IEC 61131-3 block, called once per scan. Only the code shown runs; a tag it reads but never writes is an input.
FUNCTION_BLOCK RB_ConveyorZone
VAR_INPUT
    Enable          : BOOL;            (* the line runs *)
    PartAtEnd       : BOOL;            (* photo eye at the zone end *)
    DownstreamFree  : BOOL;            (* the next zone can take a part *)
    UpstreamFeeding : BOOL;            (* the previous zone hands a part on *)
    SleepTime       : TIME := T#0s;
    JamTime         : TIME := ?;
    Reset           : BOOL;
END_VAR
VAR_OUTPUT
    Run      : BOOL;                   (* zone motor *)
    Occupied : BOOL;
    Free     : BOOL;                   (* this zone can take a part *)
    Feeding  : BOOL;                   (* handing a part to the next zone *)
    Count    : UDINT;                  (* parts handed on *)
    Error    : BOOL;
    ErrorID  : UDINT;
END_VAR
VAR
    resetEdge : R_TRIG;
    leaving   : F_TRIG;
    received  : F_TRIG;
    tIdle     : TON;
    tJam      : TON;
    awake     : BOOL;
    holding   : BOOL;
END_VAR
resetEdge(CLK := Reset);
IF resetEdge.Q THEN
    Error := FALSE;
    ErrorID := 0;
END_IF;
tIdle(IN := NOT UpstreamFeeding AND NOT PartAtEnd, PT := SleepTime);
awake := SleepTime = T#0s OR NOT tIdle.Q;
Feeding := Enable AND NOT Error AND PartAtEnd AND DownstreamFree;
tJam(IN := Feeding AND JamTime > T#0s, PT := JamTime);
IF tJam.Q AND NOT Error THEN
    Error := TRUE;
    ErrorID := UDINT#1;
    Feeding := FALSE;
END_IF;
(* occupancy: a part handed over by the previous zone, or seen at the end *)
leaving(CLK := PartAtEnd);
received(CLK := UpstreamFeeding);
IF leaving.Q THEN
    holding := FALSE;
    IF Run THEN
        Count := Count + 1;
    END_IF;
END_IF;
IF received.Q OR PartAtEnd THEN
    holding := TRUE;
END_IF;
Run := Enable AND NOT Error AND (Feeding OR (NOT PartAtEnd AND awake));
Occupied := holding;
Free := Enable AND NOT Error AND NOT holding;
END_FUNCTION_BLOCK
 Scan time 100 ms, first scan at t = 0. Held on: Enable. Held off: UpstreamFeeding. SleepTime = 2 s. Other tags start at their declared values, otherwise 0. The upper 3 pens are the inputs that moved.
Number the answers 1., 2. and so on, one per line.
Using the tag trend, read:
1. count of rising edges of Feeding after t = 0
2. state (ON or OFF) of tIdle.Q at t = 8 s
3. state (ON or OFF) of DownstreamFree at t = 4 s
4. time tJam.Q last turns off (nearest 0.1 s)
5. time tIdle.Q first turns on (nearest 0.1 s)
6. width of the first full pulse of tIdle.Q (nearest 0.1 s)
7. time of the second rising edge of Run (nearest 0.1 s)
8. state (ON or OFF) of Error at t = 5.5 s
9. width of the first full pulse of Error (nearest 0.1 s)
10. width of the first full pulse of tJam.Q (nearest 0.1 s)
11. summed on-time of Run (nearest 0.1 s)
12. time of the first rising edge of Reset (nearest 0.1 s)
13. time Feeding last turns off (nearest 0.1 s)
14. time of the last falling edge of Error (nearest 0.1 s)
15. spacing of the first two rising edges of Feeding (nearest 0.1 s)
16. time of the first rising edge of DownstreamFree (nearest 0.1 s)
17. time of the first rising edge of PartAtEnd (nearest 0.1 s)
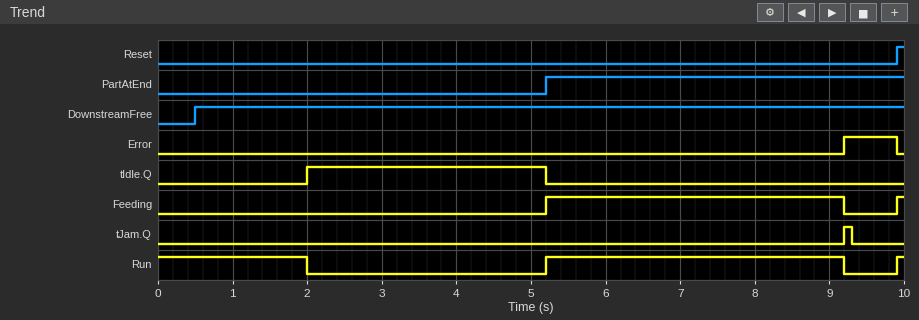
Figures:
1. 2
2. OFF
3. ON
4. 9.3 s
5. 2.0 s
6. 3.2 s
7. 9.9 s
8. OFF
9. 0.7 s
10. 0.1 s
11. 6.1 s
12. 9.9 s
13. 9.2 s
14. 9.9 s
15. 4.7 s
16. 0.5 s
17. 5.2 s
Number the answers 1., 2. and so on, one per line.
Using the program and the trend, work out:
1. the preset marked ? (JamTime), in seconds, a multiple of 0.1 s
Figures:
1. 4.0 s
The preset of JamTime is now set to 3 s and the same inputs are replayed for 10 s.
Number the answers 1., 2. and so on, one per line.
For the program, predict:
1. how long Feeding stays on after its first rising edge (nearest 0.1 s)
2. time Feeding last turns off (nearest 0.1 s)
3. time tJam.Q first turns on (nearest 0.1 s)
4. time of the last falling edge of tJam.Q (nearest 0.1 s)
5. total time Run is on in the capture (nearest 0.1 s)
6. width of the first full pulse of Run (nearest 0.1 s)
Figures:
1. 3.0 s
2. 8.2 s
3. 8.2 s
4. 8.3 s
5. 5.1 s
6. 3.0 s
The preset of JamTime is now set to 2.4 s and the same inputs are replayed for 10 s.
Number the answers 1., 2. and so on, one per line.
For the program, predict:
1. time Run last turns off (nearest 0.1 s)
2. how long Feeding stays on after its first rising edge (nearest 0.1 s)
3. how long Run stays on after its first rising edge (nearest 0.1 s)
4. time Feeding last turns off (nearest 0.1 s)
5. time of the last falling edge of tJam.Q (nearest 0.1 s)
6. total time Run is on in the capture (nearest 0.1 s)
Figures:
1. 7.6 s
2. 2.4 s
3. 2.4 s
4. 7.6 s
5. 7.7 s
6. 4.5 s
